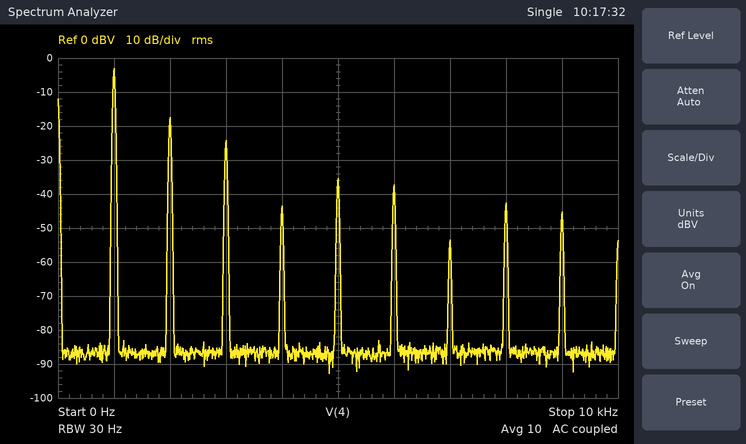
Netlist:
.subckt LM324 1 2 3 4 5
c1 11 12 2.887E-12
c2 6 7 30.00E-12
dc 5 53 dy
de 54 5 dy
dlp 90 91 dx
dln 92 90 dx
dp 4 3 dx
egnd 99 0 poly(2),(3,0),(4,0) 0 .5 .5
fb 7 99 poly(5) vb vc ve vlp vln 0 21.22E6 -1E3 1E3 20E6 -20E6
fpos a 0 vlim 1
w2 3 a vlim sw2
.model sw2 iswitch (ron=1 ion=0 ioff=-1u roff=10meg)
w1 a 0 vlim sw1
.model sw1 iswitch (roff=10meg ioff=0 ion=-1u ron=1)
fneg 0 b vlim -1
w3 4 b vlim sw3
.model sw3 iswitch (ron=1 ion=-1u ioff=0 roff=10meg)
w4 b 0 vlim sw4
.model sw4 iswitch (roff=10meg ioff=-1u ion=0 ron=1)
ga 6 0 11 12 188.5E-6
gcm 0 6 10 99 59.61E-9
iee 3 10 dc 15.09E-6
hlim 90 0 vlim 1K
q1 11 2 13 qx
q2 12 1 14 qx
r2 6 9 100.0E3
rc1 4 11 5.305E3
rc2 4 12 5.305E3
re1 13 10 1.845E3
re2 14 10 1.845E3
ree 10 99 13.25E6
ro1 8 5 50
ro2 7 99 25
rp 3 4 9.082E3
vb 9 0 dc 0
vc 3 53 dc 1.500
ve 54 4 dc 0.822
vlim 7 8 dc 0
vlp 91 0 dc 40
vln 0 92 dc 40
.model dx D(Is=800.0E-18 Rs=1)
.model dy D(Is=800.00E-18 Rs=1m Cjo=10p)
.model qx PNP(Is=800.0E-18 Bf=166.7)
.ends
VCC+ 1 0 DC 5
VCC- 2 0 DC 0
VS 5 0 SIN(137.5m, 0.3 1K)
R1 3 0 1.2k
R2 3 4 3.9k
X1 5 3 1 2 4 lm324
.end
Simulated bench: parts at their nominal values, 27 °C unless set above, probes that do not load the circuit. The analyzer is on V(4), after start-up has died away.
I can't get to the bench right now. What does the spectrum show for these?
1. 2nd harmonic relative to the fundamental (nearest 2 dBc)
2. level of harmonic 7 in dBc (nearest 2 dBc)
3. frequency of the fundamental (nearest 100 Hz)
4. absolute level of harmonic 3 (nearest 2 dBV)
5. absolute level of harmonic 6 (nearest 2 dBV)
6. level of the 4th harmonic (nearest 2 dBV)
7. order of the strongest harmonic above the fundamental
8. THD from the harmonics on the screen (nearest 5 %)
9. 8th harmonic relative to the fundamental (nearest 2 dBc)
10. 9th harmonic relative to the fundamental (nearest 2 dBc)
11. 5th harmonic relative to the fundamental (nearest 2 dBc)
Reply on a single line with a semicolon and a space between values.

-14 dBc; -50 dBc; 1.0 kHz; -24 dBV; -38 dBV; -44 dBV; 2; 20 %; -40 dBc; -42 dBc; -32 dBc
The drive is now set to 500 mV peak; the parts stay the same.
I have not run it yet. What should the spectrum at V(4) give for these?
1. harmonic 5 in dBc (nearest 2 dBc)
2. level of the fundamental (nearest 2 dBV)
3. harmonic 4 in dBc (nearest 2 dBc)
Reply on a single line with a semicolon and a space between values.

-28 dBc; 0 dBV; -30 dBc
